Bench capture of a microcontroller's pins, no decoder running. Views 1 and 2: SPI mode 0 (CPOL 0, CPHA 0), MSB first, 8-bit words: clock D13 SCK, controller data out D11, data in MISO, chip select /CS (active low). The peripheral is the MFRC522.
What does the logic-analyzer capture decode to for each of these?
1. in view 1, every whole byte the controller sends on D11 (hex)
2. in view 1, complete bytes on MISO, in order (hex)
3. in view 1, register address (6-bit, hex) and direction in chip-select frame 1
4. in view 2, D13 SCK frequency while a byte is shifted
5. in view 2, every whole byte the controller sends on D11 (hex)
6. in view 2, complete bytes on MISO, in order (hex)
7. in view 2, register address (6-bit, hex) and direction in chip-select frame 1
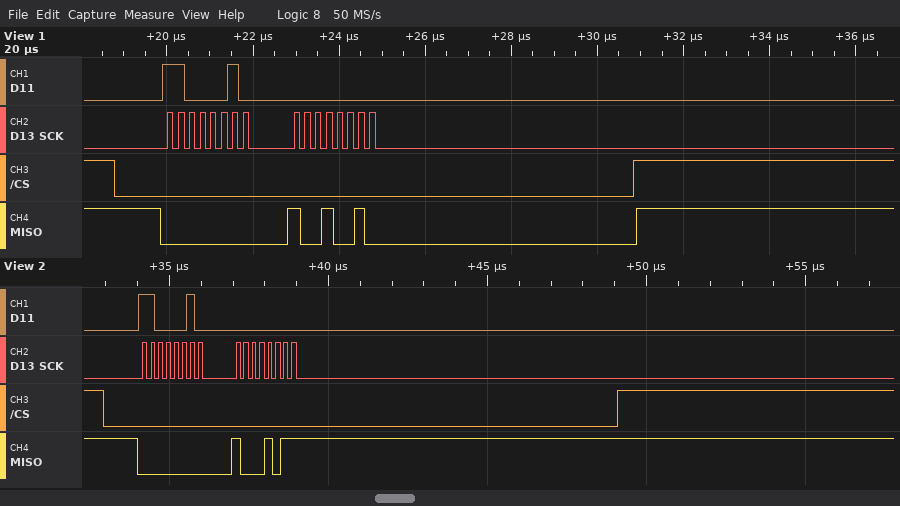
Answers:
C2 00
00 92
0x21 read
4 MHz
0xC2 0x00
0x00 0x8B
0x21 read
